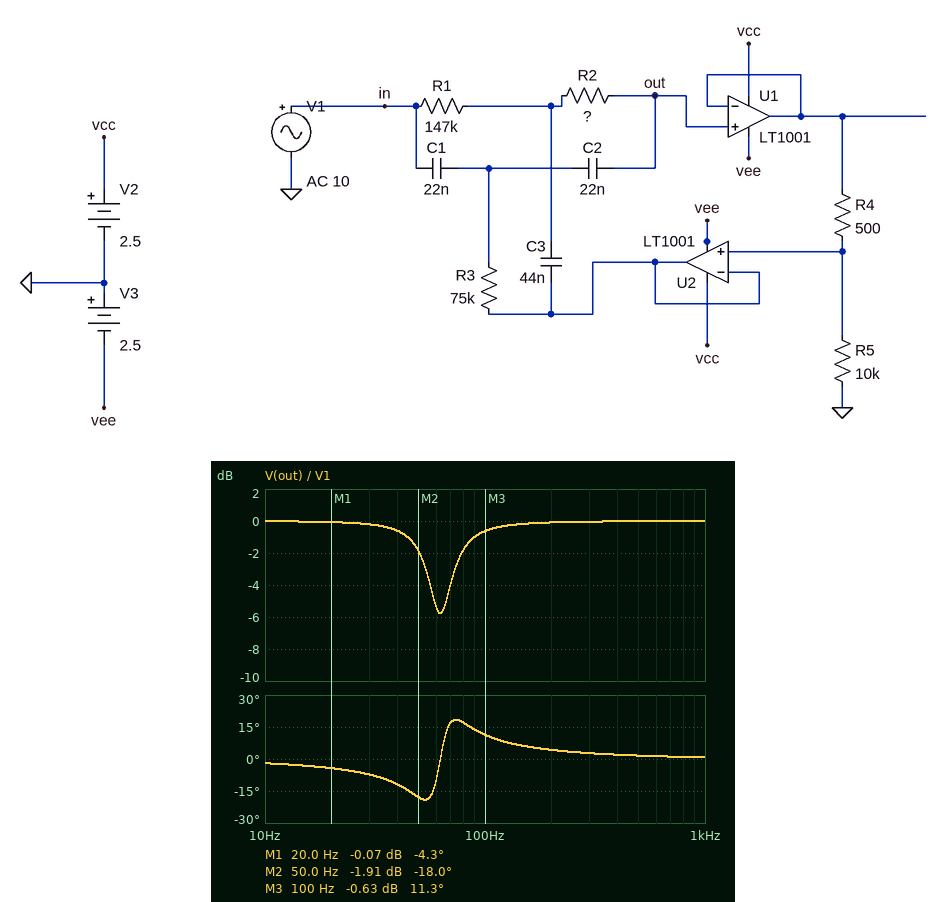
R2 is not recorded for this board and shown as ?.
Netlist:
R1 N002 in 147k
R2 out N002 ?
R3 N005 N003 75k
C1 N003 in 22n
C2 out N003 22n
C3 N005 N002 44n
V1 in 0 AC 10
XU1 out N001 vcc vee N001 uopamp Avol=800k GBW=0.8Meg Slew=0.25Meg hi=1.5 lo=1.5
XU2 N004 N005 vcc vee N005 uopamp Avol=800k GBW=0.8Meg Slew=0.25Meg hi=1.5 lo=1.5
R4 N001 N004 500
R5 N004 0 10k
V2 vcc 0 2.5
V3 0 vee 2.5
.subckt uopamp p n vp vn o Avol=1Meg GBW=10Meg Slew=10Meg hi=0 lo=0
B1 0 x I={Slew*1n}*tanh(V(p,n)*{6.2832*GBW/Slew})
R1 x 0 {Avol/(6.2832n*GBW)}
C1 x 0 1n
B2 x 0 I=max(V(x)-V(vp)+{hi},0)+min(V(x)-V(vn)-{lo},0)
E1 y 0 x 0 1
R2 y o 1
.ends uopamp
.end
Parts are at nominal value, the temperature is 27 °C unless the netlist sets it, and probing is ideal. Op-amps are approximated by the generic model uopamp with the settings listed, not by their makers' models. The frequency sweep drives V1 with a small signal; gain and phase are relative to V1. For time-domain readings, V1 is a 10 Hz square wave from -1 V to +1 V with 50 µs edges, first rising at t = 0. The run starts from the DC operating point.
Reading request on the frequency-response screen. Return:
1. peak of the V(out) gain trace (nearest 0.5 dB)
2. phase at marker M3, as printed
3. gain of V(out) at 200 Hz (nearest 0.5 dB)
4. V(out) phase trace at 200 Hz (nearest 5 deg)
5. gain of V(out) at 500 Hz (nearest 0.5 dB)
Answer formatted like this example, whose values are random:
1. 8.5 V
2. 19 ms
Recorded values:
1. 0 dB
2. 11.3 deg
3. 0 dB
4. 5 deg
5. 0 dB
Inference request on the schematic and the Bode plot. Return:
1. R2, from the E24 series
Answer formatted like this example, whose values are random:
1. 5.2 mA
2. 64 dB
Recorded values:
1. 75 kΩ
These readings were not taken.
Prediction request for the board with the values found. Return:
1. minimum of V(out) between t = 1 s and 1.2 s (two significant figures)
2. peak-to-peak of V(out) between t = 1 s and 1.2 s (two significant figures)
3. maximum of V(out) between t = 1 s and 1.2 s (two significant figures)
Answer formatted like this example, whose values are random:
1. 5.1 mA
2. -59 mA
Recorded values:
1. -1.0 V
2. 2.1 V
3. 1.0 V
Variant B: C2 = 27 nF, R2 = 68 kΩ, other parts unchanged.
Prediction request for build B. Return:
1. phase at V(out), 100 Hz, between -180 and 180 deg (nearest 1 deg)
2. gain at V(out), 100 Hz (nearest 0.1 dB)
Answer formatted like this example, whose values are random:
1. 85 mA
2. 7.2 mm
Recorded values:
1. 10 deg
2. -0.7 dB
